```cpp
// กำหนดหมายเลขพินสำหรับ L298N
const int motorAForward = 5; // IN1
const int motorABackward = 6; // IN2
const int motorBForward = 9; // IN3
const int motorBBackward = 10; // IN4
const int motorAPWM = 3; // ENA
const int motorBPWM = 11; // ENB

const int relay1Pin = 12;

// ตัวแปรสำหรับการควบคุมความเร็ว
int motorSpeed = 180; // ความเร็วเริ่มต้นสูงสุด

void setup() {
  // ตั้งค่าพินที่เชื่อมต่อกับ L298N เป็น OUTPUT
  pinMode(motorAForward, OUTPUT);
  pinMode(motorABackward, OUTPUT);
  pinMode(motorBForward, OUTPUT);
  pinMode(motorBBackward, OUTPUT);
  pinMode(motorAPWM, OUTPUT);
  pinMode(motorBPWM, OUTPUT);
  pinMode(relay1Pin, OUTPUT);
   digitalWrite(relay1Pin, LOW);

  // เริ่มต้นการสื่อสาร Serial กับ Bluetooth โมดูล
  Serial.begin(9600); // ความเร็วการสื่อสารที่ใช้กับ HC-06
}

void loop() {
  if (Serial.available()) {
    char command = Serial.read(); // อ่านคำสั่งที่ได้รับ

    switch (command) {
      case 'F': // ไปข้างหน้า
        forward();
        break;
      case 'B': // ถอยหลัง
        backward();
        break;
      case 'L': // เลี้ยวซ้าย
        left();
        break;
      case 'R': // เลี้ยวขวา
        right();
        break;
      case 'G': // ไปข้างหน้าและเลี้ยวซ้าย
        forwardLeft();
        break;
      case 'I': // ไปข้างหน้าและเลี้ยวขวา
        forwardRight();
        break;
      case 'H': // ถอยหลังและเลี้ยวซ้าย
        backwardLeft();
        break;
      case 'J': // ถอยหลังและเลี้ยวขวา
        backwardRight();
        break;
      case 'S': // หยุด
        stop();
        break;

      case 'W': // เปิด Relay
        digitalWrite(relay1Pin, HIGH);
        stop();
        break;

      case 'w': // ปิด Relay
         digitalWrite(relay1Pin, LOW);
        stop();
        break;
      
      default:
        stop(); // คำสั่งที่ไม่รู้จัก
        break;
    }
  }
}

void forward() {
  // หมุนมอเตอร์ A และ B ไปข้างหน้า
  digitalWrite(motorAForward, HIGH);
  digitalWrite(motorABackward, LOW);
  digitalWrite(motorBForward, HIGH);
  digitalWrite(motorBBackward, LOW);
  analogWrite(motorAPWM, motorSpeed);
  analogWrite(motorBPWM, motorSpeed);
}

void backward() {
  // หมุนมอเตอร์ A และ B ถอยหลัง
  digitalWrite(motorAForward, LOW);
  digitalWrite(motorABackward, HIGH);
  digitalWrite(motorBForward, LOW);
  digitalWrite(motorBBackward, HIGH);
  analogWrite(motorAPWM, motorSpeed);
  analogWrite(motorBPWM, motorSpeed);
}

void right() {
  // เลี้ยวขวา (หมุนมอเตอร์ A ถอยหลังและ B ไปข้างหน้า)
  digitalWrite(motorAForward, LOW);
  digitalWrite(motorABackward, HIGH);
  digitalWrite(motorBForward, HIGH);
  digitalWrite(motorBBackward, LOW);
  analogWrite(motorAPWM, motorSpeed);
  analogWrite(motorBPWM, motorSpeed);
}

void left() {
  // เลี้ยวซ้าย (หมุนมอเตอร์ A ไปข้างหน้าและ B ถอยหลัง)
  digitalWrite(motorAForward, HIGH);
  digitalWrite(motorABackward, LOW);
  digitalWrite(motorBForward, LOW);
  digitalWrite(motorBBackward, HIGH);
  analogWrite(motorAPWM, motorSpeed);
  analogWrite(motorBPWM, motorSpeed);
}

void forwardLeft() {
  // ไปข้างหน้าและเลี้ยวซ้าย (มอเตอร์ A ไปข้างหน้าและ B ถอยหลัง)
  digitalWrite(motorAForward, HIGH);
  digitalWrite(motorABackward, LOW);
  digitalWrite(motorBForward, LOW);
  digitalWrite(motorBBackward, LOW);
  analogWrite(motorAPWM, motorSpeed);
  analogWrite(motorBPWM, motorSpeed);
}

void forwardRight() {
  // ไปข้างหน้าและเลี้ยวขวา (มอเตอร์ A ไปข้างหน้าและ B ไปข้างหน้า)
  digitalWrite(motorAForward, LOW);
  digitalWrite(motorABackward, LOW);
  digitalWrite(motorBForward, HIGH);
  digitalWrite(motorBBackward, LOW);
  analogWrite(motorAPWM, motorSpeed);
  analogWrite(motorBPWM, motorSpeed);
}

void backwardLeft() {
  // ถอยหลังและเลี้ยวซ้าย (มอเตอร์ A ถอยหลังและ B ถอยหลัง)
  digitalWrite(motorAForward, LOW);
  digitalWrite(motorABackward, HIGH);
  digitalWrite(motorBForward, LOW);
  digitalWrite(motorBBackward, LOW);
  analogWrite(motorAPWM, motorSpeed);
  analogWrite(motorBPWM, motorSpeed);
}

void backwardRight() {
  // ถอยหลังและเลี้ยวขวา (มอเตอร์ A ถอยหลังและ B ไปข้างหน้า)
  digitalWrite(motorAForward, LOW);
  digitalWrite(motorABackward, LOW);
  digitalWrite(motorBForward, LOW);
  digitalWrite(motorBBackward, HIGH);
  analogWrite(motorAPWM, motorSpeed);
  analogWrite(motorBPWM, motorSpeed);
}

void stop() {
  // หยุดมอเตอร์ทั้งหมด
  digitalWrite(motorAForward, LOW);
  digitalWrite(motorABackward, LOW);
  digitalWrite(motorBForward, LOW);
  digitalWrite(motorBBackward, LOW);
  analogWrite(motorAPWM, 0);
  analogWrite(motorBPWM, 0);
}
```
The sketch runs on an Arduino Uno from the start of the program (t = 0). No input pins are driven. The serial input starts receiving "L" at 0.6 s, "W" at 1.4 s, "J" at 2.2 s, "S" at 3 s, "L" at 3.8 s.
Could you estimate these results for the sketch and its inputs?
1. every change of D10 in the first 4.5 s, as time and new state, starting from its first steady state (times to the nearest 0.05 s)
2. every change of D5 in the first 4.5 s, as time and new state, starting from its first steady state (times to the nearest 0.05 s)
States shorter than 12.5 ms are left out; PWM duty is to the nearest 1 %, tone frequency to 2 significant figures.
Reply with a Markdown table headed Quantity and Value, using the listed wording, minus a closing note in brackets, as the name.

| Quantity | Value |
|---|---|
| every change of D10 in the first 4.5 s, as time and new state, starting from its first steady state | 0 s low; 0.6 s high; 1.4 s low; 2.2 s high; 3 s low; 3.8 s high |
| every change of D5 in the first 4.5 s, as time and new state, starting from its first steady state | 0 s low; 0.6 s high; 1.4 s low; 3.8 s high |
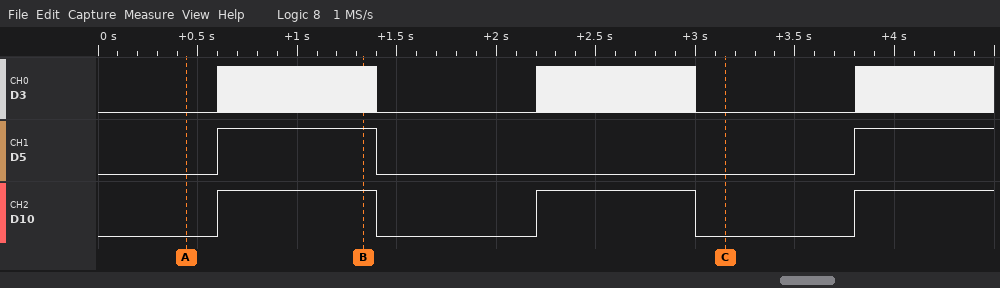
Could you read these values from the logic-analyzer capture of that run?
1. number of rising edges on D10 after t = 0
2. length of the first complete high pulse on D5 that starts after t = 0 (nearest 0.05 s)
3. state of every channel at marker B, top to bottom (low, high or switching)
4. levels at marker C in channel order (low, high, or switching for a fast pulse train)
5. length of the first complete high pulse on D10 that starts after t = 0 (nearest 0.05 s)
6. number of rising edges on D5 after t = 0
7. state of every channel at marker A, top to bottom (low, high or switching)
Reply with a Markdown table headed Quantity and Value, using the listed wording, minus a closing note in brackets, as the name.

| Quantity | Value |
|---|---|
| number of rising edges on D10 after t = 0 | 3 |
| length of the first complete high pulse on D5 that starts after t = 0 | 0.80 s |
| state of every channel at marker B, top to bottom | D3 switching, D5 high, D10 high |
| levels at marker C in channel order | D3 low, D5 low, D10 low |
| length of the first complete high pulse on D10 that starts after t = 0 | 0.80 s |
| number of rising edges on D5 after t = 0 | 2 |
| state of every channel at marker A, top to bottom | D3 low, D5 low, D10 low |
